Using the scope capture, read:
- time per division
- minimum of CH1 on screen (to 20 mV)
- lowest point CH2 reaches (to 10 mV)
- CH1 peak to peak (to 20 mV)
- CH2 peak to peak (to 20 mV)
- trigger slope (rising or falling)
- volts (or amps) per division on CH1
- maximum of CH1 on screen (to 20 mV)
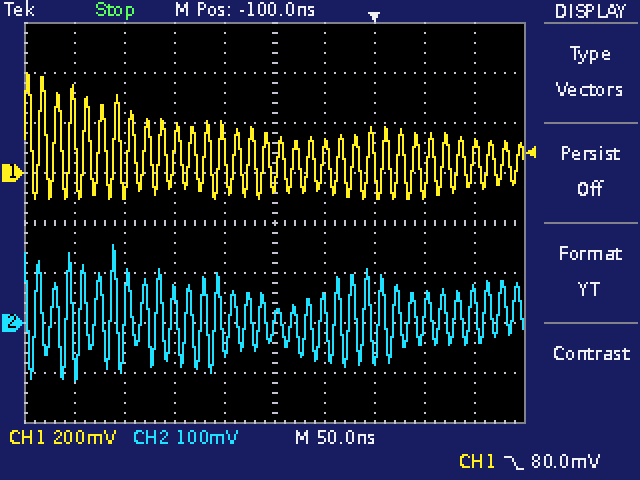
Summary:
50 ns
-100 mV
-120 mV
500 mV
280 mV
falling
200 mV
400 mV
